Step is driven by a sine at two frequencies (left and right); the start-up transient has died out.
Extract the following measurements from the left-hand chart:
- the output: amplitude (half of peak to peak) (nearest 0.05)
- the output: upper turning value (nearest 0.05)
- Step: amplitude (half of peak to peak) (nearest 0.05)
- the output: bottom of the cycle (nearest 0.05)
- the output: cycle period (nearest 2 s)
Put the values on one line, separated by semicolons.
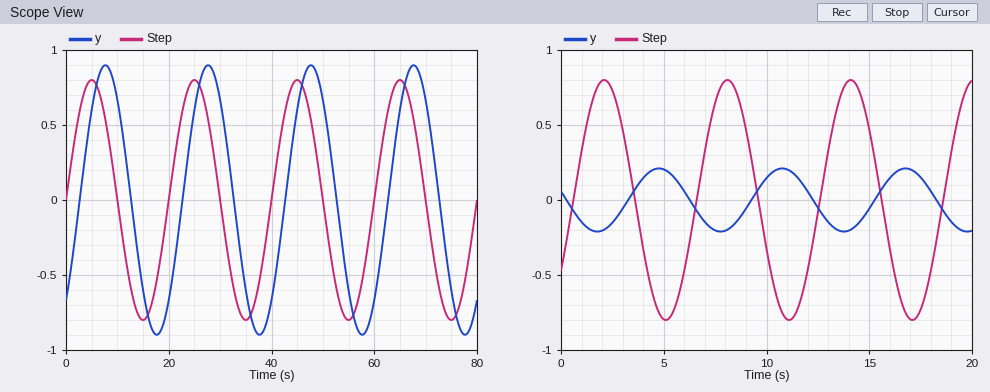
0.90; 0.90; 0.80; -0.90; 20 s
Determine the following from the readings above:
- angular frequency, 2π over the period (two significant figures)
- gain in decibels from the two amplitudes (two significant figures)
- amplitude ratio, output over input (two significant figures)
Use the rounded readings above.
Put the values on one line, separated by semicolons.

0.31 rad/s; 1.0 dB; 1.1
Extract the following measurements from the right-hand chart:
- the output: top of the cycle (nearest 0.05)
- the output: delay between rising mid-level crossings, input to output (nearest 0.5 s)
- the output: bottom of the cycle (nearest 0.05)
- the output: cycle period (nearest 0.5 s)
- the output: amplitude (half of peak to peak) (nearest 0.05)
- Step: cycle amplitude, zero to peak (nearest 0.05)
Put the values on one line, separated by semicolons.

0.20; 2.5 s; -0.20; 6.0 s; 0.20; 0.80
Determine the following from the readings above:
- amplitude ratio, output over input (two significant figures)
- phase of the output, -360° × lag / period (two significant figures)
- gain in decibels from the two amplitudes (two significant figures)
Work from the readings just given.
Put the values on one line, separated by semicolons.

0.25; -150°; -12 dB
